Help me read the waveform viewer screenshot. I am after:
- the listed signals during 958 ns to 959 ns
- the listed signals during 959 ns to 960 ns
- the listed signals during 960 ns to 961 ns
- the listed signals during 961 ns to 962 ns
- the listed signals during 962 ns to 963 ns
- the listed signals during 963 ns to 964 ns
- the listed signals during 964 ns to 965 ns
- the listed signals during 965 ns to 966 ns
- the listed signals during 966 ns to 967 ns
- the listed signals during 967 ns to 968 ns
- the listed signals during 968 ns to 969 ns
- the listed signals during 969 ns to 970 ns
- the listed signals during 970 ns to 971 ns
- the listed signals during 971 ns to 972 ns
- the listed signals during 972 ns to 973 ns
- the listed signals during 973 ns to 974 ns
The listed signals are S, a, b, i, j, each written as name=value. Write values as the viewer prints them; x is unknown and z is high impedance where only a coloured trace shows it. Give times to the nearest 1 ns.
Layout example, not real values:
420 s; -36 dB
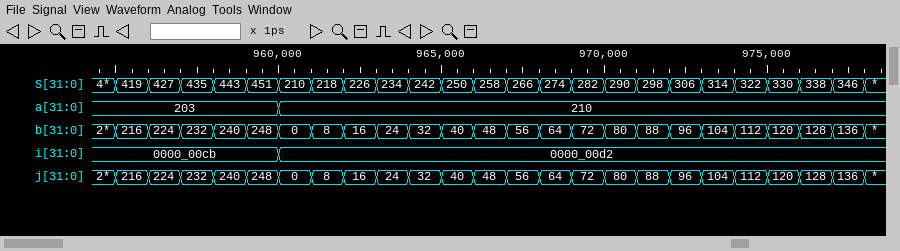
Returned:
S=443, a=203, b=240, i=0000_00cb, j=240; S=451, a=203, b=248, i=0000_00cb, j=248; S=210, a=210, b=0, i=0000_00d2, j=0; S=218, a=210, b=8, i=0000_00d2, j=8; S=226, a=210, b=16, i=0000_00d2, j=16; S=234, a=210, b=24, i=0000_00d2, j=24; S=242, a=210, b=32, i=0000_00d2, j=32; S=250, a=210, b=40, i=0000_00d2, j=40; S=258, a=210, b=48, i=0000_00d2, j=48; S=266, a=210, b=56, i=0000_00d2, j=56; S=274, a=210, b=64, i=0000_00d2, j=64; S=282, a=210, b=72, i=0000_00d2, j=72; S=290, a=210, b=80, i=0000_00d2, j=80; S=298, a=210, b=88, i=0000_00d2, j=88; S=306, a=210, b=96, i=0000_00d2, j=96; S=314, a=210, b=104, i=0000_00d2, j=104
